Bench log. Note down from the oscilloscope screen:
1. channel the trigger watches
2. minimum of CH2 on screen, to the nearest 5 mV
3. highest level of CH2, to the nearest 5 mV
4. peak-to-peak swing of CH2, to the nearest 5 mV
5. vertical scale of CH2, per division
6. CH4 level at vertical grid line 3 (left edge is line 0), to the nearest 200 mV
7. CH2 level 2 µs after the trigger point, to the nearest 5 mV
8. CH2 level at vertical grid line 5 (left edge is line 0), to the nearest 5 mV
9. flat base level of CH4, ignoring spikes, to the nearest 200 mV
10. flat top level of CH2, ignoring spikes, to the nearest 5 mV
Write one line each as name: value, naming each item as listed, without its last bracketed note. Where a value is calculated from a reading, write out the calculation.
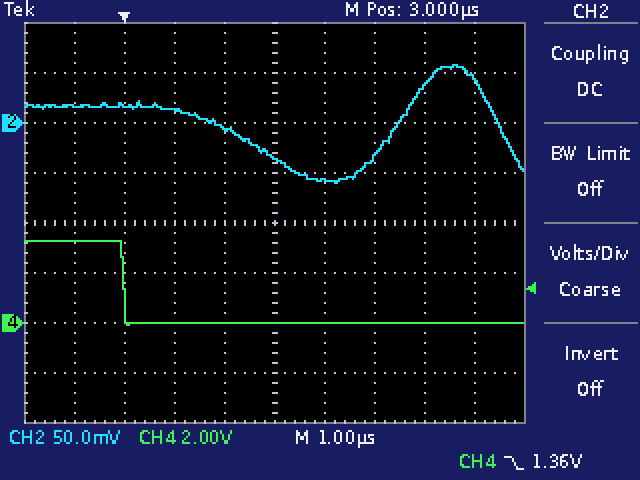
channel the trigger watches: CH4
minimum of CH2 on screen, to the nearest 5 mV: -60 mV
highest level of CH2, to the nearest 5 mV: 60 mV
peak-to-peak swing of CH2, to the nearest 5 mV: 60 mV − (-60 mV) = 120 mV
vertical scale of CH2, per division: 50 mV
CH4 level at vertical grid line 3 (left edge is line 0), to the nearest 200 mV: 0.0 V
CH2 level 2 µs after the trigger point, to the nearest 5 mV: -5 mV
CH2 level at vertical grid line 5 (left edge is line 0), to the nearest 5 mV: -35 mV
flat base level of CH4, ignoring spikes, to the nearest 200 mV: 0.0 V
flat top level of CH2, ignoring spikes, to the nearest 5 mV: 15 mV
